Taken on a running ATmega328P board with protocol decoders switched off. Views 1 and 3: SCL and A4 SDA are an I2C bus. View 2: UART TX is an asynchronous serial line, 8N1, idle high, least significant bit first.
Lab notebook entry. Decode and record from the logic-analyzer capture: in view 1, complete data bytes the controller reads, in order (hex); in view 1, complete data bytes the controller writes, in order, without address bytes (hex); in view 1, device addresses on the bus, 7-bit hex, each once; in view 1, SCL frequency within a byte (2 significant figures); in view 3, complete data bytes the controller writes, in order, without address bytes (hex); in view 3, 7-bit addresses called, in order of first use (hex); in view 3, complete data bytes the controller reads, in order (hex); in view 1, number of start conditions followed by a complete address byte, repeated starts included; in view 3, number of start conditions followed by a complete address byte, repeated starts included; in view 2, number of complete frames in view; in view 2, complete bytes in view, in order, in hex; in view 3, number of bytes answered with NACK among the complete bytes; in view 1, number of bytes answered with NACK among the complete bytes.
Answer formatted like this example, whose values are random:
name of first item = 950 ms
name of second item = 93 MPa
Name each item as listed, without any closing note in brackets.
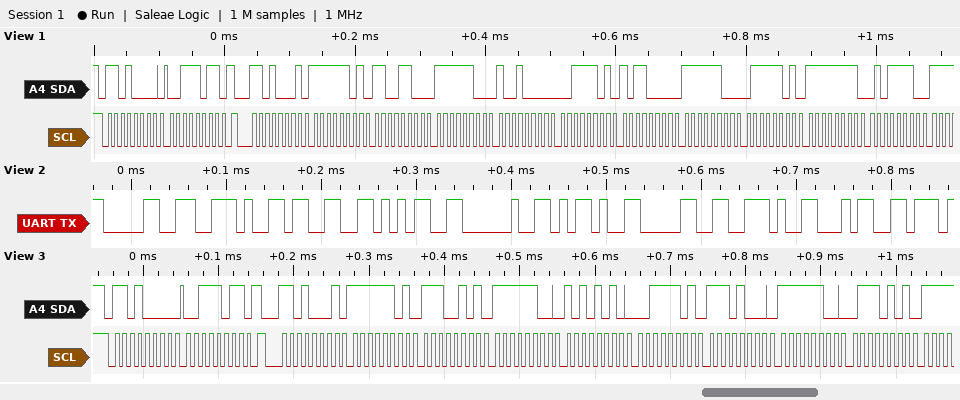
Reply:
in view 1, complete data bytes the controller reads, in order = FD CC FC 90 3D B0 FC 7D FF 5E
in view 1, complete data bytes the controller writes, in order, without address bytes = 3B
in view 1, device addresses on the bus, 7-bit hex, each once = 0x68
in view 1, SCL frequency within a byte = 100 kHz
in view 3, complete data bytes the controller writes, in order, without address bytes = 3B
in view 3, 7-bit addresses called, in order of first use = 0x68
in view 3, complete data bytes the controller reads, in order = FD E5 FC AA 3D E8 FC 75
in view 1, number of start conditions followed by a complete address byte, repeated starts included = 2
in view 3, number of start conditions followed by a complete address byte, repeated starts included = 2
in view 2, number of complete frames in view = 9
in view 2, complete bytes in view, in order, in hex = 30 2E 33 35 20 2D 30 2E 34
in view 3, number of bytes answered with NACK among the complete bytes = 0
in view 1, number of bytes answered with NACK among the complete bytes = 0
